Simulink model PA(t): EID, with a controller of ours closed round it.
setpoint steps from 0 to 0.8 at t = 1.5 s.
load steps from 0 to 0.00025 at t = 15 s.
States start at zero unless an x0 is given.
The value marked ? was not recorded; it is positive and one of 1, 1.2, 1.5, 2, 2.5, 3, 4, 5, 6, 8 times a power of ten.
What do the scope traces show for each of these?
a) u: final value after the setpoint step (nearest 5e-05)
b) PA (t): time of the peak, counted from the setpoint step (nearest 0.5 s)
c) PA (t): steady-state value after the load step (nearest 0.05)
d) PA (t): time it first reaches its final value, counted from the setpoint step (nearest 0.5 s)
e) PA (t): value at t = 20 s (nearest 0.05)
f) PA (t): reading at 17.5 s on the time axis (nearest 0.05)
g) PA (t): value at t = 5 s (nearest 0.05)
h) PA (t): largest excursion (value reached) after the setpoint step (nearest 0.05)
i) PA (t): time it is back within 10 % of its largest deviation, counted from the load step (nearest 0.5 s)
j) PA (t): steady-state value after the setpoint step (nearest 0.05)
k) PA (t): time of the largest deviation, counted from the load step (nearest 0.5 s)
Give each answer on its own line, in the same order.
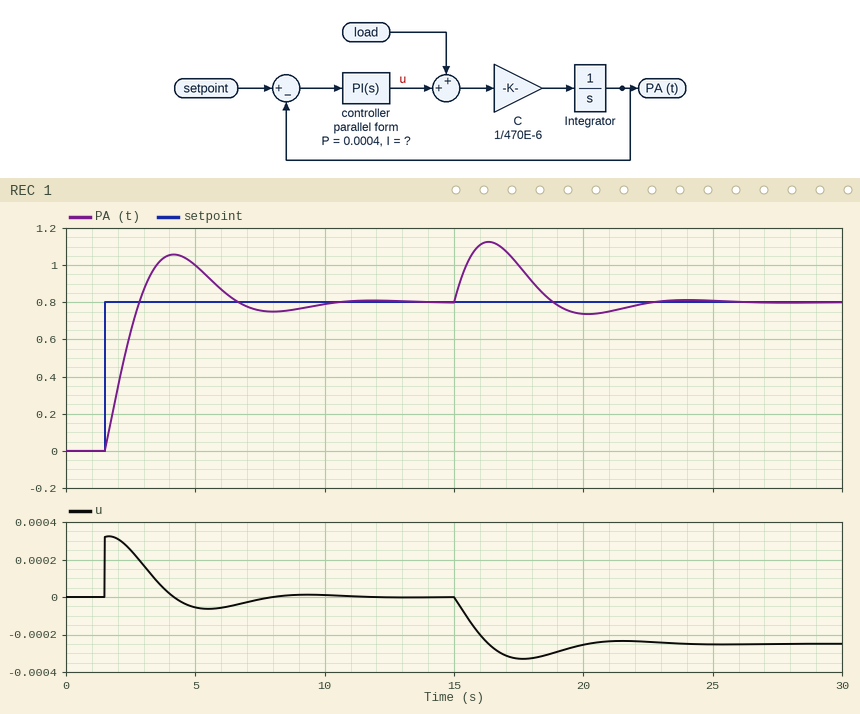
0.00000
2.5 s
0.80
1.5 s
0.75
1.00
1.00
1.05
6.5 s
0.80
1.5 s
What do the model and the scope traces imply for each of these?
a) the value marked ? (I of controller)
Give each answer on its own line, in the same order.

0.0004
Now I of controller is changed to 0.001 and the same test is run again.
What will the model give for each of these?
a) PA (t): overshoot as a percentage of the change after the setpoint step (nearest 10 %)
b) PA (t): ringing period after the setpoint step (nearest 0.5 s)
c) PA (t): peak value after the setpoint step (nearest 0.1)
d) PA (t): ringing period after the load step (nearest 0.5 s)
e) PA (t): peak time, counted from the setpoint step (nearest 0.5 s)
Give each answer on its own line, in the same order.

50 %
4.5 s
1.2
4.5 s
2.0 s
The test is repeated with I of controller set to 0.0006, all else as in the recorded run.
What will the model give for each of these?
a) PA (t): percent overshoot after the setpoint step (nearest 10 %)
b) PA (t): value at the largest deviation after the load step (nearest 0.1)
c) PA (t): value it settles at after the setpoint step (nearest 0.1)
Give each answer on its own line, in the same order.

40 %
1.1
0.8
